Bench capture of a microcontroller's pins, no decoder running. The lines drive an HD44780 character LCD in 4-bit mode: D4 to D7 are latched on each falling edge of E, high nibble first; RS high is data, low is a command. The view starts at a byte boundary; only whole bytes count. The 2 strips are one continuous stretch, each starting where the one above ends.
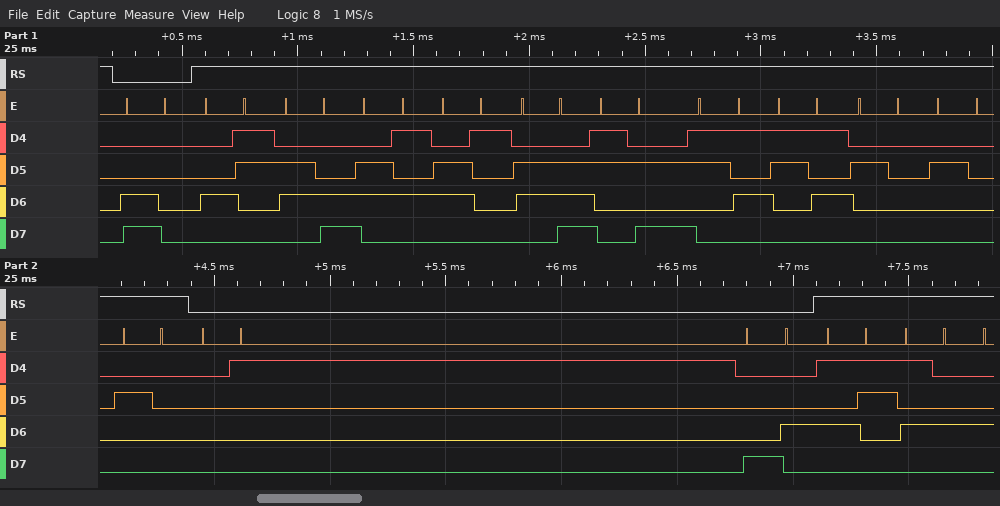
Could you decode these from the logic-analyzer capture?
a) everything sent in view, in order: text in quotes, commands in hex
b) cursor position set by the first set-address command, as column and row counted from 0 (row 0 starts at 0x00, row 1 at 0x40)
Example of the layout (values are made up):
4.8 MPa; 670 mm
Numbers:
0xC0 "Clean:55   " 0x01 0x84 "ST"; column 0, row 1
